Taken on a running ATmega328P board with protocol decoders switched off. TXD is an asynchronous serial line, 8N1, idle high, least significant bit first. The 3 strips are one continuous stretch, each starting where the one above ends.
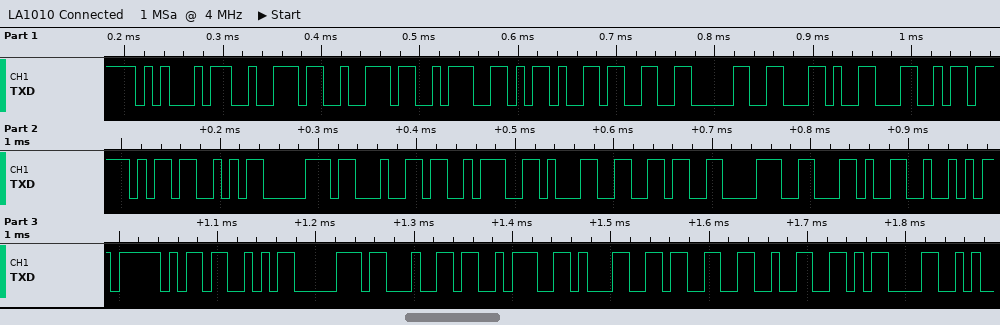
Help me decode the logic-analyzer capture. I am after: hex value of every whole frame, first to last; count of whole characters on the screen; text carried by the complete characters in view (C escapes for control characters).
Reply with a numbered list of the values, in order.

1. 0x45 0x72 0x72 0x3A 0x2D 0x33 0x30 0x2C 0x4C 0x5F 0x53 0x70 0x64 0x3A 0x31 0x36 0x38 0x2C 0x52 0x5F 0x53 0x70 0x64 0x3A 0x31 0x33 0x32 0x0D
2. 28
3. "Err:-30,L_Spd:168,R_Spd:132\r"
